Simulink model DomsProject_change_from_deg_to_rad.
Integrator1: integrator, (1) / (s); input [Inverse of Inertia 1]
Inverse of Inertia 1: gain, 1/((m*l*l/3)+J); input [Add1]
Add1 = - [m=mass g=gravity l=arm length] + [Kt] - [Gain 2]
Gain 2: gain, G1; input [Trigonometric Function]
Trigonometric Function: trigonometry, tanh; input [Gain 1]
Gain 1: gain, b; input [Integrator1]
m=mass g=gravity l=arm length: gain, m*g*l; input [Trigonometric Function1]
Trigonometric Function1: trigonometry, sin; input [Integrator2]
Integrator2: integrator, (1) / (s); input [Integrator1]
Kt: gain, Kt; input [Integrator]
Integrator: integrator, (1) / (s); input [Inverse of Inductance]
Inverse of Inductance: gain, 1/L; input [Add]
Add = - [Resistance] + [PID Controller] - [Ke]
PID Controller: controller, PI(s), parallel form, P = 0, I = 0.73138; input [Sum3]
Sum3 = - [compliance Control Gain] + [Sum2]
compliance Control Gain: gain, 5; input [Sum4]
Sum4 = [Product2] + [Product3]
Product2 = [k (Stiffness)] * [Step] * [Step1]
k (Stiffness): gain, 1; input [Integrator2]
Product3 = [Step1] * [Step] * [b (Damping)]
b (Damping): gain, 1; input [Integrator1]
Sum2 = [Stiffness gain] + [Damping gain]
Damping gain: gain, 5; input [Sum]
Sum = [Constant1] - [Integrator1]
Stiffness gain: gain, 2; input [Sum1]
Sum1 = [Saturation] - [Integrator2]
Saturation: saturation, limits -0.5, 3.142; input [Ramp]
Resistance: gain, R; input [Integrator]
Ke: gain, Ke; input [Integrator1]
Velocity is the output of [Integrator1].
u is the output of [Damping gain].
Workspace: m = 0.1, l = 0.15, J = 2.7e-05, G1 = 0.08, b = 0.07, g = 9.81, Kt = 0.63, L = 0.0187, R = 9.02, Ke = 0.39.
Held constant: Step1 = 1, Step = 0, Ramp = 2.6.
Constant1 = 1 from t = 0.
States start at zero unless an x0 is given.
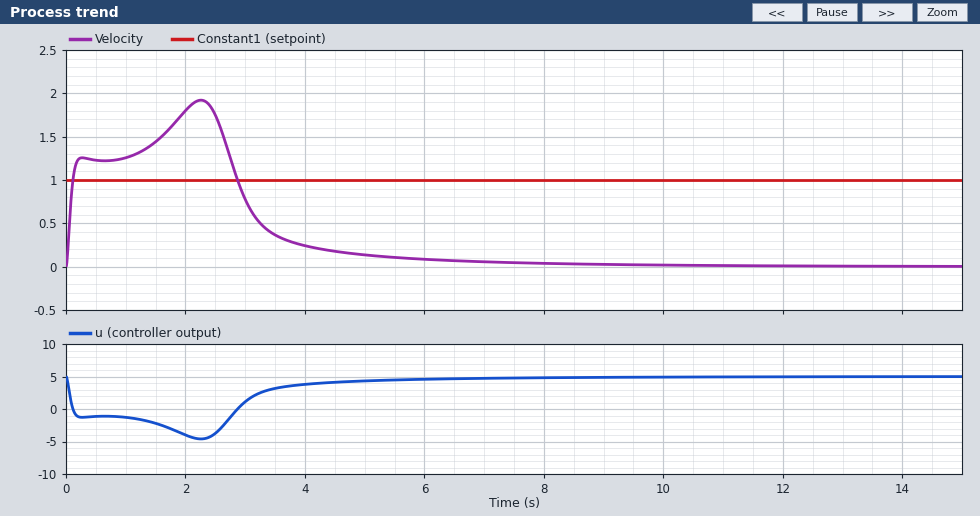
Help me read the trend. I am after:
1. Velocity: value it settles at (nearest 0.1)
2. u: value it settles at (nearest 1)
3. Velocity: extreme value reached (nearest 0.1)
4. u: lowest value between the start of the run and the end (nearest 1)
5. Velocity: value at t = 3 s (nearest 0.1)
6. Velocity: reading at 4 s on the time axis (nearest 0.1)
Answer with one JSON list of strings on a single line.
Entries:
["0.0", "5", "1.9", "-5", "0.8", "0.2"]
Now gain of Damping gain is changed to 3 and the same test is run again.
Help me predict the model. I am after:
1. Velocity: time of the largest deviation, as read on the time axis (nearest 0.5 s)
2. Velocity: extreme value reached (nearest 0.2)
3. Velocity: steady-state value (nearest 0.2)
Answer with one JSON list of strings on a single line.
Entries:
["2.0 s", "3.2", "0.0"]
